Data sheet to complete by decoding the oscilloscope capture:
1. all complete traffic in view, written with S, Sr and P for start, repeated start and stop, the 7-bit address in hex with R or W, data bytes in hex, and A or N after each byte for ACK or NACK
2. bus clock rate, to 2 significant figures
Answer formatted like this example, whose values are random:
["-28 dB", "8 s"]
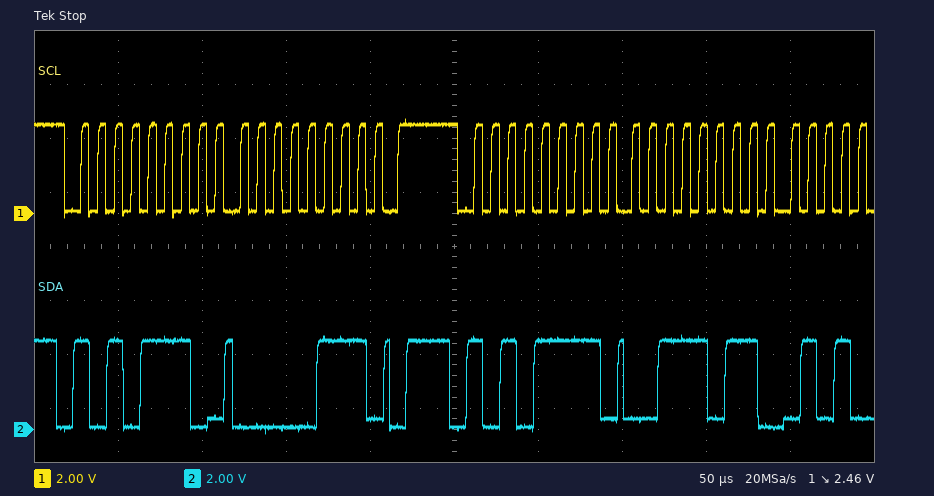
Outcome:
["S 57W A 07 A P S 57R A 3B A", "100 kHz"]
